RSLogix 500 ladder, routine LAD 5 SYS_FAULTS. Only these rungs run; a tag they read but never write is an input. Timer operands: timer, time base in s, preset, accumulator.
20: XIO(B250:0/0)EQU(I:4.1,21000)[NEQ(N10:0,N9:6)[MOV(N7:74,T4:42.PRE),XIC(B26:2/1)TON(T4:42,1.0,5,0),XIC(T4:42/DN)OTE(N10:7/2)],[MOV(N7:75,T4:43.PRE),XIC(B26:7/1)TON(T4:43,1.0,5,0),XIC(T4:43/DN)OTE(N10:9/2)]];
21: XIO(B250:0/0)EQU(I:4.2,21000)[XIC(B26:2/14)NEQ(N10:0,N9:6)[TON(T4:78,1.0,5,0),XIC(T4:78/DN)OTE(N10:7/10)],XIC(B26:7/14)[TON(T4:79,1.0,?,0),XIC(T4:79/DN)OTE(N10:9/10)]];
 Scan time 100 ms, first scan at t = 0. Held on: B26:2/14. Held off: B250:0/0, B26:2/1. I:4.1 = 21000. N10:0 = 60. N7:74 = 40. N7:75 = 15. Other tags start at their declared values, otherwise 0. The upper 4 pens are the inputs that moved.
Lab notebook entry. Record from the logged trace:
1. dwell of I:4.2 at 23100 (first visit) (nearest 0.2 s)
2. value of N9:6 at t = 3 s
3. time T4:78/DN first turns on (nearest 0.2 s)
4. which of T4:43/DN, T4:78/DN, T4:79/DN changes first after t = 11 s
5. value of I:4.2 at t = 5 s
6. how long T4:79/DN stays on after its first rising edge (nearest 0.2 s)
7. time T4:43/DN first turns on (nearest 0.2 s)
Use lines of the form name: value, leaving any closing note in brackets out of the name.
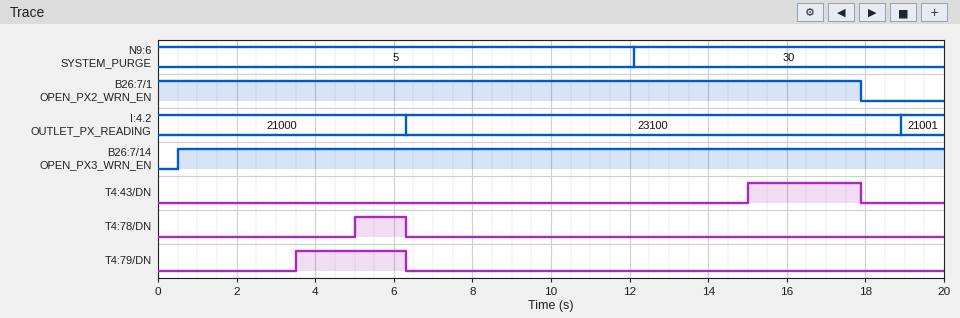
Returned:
dwell of I:4.2 at 23100 (first visit): 12.6 s
value of N9:6 at t = 3 s: 5
time T4:78/DN first turns on: 5.0 s
which of T4:43/DN, T4:78/DN, T4:79/DN changes first after t = 11 s: T4:43/DN
value of I:4.2 at t = 5 s: 21000
how long T4:79/DN stays on after its first rising edge: 2.8 s
time T4:43/DN first turns on: 15.0 s
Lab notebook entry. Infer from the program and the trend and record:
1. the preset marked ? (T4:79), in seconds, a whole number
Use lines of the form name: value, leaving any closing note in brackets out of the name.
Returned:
the preset marked ? (T4:79), in seconds, a whole number: 3 s
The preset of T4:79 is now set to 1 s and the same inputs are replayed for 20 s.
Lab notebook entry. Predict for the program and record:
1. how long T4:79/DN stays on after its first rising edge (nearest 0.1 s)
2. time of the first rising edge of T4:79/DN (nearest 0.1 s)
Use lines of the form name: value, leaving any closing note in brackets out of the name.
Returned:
how long T4:79/DN stays on after its first rising edge: 4.8 s
time of the first rising edge of T4:79/DN: 1.5 s
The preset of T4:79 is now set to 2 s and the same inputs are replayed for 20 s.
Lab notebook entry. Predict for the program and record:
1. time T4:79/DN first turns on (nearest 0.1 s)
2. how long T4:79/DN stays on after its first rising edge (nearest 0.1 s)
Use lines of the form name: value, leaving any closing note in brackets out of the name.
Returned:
time T4:79/DN first turns on: 2.5 s
how long T4:79/DN stays on after its first rising edge: 3.8 s
